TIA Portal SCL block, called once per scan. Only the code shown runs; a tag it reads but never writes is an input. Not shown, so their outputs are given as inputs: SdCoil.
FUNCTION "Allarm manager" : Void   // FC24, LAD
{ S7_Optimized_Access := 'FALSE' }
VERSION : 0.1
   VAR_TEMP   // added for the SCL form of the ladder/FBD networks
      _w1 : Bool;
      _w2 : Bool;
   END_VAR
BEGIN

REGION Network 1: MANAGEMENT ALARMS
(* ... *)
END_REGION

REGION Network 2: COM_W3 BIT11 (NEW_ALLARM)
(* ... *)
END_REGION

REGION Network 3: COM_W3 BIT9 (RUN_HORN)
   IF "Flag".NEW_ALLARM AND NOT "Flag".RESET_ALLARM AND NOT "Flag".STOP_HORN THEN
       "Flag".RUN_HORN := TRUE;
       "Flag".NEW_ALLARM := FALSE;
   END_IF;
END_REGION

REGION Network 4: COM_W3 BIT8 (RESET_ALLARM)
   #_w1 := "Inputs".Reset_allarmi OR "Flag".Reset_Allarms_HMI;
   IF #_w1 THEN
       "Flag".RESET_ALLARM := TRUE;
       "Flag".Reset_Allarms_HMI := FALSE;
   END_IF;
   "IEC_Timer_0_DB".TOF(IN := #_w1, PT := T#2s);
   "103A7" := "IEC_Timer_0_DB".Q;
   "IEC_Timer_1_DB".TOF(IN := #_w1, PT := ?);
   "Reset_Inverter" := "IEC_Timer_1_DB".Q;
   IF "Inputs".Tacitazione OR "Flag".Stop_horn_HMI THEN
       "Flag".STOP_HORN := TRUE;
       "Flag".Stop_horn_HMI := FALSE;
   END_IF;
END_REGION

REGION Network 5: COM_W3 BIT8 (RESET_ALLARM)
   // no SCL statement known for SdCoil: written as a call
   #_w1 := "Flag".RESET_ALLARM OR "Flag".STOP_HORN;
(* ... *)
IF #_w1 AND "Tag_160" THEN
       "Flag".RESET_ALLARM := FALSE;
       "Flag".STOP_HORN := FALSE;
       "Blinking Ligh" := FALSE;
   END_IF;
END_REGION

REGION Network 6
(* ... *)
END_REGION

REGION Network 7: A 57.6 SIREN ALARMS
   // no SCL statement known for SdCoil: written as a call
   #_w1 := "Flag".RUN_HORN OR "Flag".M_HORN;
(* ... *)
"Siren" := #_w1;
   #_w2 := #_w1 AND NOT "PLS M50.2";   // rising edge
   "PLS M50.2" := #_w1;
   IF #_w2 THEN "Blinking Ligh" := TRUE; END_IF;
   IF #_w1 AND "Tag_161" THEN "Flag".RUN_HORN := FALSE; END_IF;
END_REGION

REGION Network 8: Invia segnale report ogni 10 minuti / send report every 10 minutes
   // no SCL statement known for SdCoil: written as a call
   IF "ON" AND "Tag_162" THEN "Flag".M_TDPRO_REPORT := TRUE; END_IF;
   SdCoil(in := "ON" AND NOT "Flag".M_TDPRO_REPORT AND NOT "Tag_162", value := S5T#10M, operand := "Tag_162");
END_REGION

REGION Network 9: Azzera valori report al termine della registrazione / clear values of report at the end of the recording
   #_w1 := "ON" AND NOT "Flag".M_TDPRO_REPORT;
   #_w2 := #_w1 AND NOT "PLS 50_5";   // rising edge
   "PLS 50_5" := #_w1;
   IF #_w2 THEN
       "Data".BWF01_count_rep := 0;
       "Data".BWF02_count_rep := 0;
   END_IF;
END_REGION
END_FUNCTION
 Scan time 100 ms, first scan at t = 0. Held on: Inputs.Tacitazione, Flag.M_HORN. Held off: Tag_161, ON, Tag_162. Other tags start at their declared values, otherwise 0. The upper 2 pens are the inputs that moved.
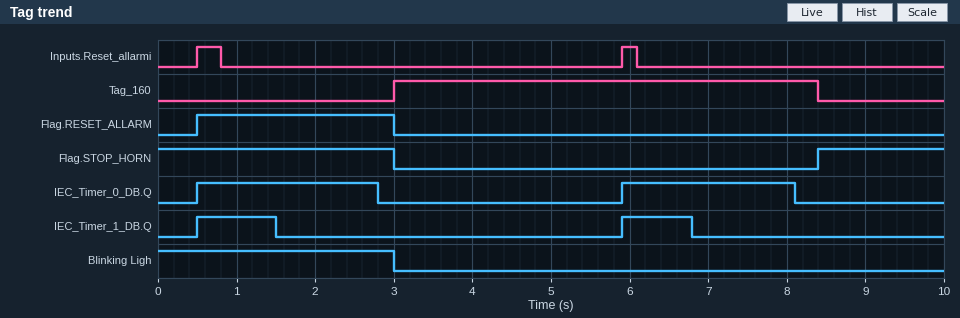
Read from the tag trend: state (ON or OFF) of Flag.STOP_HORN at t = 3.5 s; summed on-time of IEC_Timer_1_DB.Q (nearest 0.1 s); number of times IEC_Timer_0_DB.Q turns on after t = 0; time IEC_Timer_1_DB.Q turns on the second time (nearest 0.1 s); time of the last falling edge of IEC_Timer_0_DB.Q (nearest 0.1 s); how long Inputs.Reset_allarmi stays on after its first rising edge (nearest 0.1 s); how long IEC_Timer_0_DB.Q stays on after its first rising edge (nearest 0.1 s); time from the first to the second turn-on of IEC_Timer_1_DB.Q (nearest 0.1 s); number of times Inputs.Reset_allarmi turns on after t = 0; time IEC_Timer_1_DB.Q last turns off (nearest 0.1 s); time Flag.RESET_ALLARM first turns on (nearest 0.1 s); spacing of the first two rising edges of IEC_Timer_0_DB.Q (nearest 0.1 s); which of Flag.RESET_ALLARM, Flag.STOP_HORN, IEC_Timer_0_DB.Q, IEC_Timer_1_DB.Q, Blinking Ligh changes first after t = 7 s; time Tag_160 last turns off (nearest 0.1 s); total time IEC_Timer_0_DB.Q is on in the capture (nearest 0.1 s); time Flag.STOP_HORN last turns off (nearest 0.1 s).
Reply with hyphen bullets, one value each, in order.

- OFF
- 1.9 s
- 2
- 5.9 s
- 8.1 s
- 0.3 s
- 2.3 s
- 5.4 s
- 2
- 6.8 s
- 0.5 s
- 5.4 s
- IEC_Timer_0_DB.Q
- 8.4 s
- 4.5 s
- 3.0 s
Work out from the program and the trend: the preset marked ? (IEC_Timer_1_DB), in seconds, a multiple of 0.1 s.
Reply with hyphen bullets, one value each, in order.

- 0.7 s
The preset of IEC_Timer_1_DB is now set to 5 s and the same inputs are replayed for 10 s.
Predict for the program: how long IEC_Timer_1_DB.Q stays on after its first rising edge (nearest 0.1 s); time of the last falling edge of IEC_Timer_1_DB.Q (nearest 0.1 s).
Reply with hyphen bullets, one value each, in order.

- 5.3 s
- 5.8 s
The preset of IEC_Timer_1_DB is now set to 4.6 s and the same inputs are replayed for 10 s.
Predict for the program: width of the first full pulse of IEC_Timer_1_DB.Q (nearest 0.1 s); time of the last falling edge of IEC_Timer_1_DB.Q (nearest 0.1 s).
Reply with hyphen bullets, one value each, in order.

- 4.9 s
- 5.4 s
